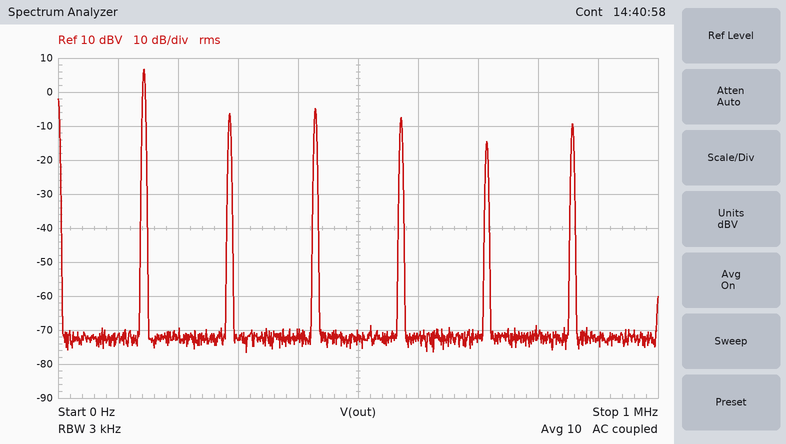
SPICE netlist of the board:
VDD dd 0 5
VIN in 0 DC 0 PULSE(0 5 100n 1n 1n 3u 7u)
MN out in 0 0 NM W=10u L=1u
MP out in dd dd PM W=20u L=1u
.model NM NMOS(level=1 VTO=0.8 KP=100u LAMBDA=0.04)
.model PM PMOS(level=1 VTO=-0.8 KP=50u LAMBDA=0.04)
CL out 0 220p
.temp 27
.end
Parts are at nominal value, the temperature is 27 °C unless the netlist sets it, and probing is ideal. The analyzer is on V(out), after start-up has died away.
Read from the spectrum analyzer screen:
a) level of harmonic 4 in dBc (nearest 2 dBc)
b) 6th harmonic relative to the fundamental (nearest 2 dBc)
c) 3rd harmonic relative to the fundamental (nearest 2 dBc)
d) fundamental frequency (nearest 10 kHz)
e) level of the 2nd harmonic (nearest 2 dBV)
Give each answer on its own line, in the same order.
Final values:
-14 dBc
-16 dBc
-12 dBc
140 kHz
-6 dBV
